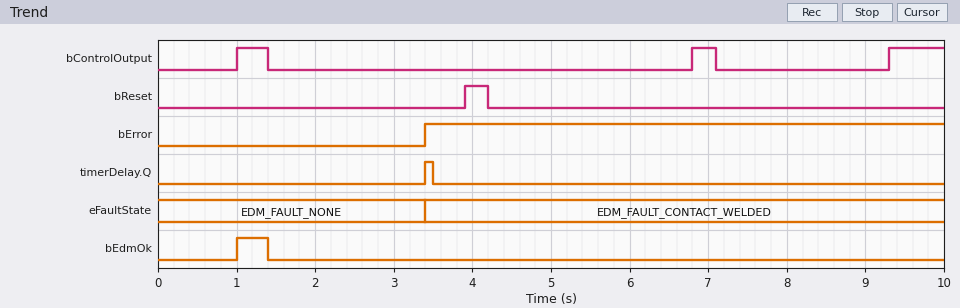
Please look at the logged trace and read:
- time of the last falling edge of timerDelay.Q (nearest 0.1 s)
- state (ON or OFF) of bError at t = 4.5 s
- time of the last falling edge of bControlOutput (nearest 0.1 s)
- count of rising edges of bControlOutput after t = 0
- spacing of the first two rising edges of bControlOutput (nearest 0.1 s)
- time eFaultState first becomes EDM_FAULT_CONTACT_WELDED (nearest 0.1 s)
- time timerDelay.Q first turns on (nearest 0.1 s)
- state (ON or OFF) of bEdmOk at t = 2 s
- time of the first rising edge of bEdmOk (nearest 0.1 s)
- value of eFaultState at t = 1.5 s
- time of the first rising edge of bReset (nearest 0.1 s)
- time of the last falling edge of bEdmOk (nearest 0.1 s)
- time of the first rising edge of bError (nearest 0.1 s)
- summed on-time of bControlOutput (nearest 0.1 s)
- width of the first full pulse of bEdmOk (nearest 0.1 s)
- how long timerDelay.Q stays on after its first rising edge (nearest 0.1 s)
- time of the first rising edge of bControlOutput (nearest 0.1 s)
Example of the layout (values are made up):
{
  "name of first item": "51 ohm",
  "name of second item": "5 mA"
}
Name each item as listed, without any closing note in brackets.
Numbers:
{
  "time of the last falling edge of timerDelay.Q": "3.5 s",
  "state (ON or OFF) of bError at t = 4.5 s": "ON",
  "time of the last falling edge of bControlOutput": "7.1 s",
  "count of rising edges of bControlOutput after t = 0": "3",
  "spacing of the first two rising edges of bControlOutput": "5.8 s",
  "time eFaultState first becomes EDM_FAULT_CONTACT_WELDED": "3.4 s",
  "time timerDelay.Q first turns on": "3.4 s",
  "state (ON or OFF) of bEdmOk at t = 2 s": "OFF",
  "time of the first rising edge of bEdmOk": "1.0 s",
  "value of eFaultState at t = 1.5 s": "EDM_FAULT_NONE",
  "time of the first rising edge of bReset": "3.9 s",
  "time of the last falling edge of bEdmOk": "1.4 s",
  "time of the first rising edge of bError": "3.4 s",
  "summed on-time of bControlOutput": "1.4 s",
  "width of the first full pulse of bEdmOk": "0.4 s",
  "how long timerDelay.Q stays on after its first rising edge": "0.1 s",
  "time of the first rising edge of bControlOutput": "1.0 s"
}
